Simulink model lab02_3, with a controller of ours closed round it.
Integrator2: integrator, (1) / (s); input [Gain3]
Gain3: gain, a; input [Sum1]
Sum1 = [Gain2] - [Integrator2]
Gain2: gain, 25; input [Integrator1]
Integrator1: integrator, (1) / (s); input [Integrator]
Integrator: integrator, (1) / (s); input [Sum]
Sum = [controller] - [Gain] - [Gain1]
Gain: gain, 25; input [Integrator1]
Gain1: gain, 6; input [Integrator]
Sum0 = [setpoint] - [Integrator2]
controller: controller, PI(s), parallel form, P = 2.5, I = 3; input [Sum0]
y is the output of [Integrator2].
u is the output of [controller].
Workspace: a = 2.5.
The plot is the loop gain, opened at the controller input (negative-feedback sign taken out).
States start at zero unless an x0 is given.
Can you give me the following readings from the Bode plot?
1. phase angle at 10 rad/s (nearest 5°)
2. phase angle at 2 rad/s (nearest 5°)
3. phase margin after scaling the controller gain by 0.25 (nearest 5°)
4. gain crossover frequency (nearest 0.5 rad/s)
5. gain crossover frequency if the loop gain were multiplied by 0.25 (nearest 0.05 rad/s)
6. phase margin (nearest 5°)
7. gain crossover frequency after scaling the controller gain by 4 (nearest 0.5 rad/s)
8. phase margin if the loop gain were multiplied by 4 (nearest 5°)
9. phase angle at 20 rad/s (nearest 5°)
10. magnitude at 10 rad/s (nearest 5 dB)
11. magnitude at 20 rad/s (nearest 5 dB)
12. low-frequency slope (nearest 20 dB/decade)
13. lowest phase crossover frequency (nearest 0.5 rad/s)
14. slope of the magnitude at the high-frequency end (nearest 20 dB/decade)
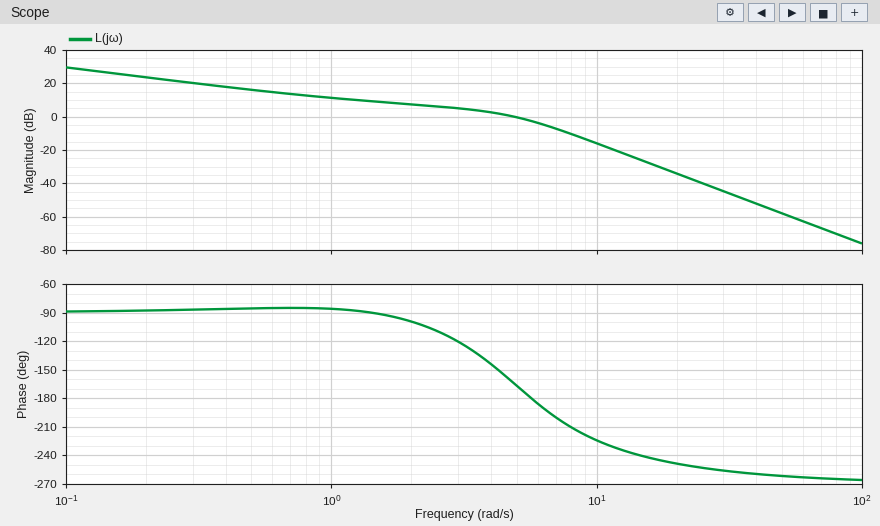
-225°
-100°
95°
5.0 rad/s
0.90 rad/s
15°
8.5 rad/s
-35°
-250°
-15 dB
-35 dB
-20 dB/decade
5.5 rad/s
-60 dB/decade
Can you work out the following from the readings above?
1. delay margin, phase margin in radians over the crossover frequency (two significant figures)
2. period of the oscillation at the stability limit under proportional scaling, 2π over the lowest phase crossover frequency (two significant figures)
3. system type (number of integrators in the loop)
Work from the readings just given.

0.052 s
1.1 s
1
